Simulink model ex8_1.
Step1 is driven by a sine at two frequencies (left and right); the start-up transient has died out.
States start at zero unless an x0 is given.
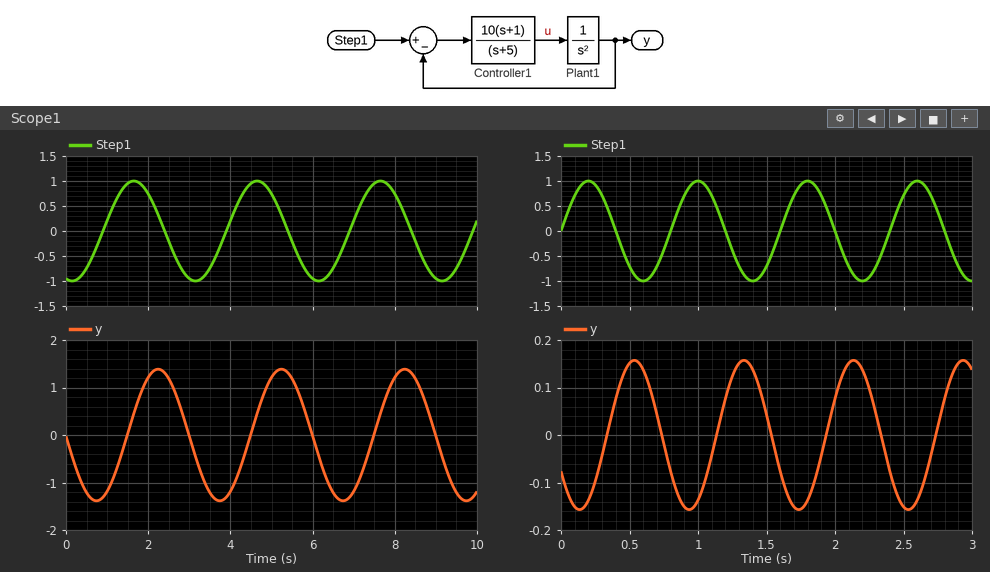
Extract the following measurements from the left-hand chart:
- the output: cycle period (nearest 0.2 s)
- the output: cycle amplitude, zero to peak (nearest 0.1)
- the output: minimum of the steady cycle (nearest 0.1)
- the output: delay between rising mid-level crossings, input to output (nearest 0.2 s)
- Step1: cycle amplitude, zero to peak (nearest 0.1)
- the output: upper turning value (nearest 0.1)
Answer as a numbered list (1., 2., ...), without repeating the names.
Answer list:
1. 3.0 s
2. 1.4
3. -1.4
4. 0.6 s
5. 1.0
6. 1.4
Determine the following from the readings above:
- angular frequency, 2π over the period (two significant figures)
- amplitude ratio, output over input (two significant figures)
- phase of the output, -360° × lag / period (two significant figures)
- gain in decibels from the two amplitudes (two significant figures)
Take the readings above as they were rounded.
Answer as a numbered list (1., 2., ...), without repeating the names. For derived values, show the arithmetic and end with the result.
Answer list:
1. 2π / 3 = 2.1 rad/s
2. 1.4 / 1 = 1.4
3. -360 × 0.6 / 3 = -72°
4. 20 log10(1.4 / 1) = 2.9 dB
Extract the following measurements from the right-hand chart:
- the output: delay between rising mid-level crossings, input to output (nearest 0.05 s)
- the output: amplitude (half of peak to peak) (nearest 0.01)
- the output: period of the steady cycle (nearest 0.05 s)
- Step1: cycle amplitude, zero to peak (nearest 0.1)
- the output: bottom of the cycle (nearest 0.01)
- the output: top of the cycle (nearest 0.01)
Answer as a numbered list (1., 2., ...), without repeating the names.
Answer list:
1. 0.35 s
2. 0.16
3. 0.80 s
4. 1.0
5. -0.16
6. 0.16
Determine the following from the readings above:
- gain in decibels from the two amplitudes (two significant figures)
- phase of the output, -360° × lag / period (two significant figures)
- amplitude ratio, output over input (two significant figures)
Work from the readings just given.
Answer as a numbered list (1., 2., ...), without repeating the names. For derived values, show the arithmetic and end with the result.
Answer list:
1. 20 log10(0.16 / 1) = -16 dB
2. -360 × 0.35 / 0.8 = -160°
3. 0.16 / 1 = 0.16
